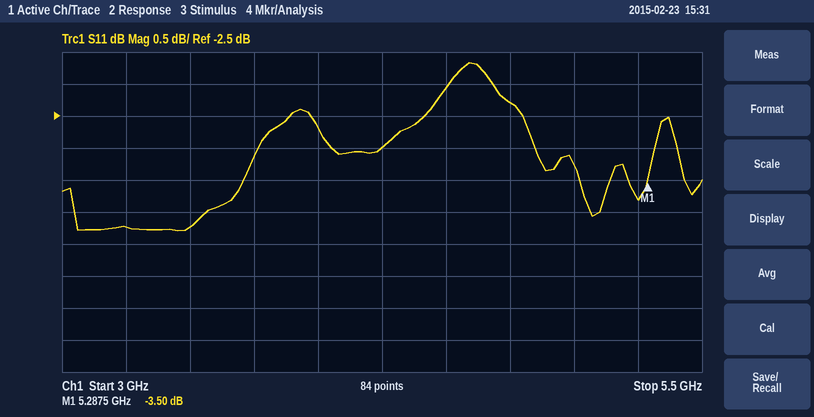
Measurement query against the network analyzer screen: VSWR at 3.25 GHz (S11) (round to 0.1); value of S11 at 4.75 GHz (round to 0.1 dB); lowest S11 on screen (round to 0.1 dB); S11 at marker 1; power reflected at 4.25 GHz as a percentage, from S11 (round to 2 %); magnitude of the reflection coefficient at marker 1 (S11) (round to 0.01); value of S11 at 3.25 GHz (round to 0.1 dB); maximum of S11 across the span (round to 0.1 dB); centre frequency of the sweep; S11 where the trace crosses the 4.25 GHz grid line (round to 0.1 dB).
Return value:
4.2
-2.3 dB
-4.3 dB
-3.50 dB
50 %
0.67
-4.2 dB
-1.7 dB
4.25 GHz
-3.0 dB
